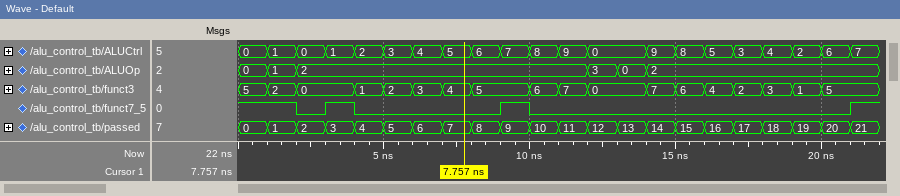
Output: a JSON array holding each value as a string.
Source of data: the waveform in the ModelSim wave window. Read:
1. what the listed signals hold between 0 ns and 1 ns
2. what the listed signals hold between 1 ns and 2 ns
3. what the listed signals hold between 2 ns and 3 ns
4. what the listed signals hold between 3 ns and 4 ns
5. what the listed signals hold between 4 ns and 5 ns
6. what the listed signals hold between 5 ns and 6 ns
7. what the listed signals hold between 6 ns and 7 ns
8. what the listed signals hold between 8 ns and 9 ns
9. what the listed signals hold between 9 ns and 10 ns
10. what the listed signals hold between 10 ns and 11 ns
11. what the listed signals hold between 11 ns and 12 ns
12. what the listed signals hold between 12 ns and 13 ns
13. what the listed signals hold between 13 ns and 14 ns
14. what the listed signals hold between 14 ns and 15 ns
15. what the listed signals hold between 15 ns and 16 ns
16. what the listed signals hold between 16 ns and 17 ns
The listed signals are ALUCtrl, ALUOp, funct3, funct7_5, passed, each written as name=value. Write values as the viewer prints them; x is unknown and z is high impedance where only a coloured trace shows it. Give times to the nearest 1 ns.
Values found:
["ALUCtrl=0, ALUOp=0, funct3=5, funct7_5=1, passed=0", "ALUCtrl=1, ALUOp=1, funct3=2, funct7_5=1, passed=1", "ALUCtrl=0, ALUOp=2, funct3=0, funct7_5=0, passed=2", "ALUCtrl=1, ALUOp=2, funct3=0, funct7_5=1, passed=3", "ALUCtrl=2, ALUOp=2, funct3=1, funct7_5=0, passed=4", "ALUCtrl=3, ALUOp=2, funct3=2, funct7_5=0, passed=5", "ALUCtrl=4, ALUOp=2, funct3=3, funct7_5=0, passed=6", "ALUCtrl=6, ALUOp=2, funct3=5, funct7_5=0, passed=8", "ALUCtrl=7, ALUOp=2, funct3=5, funct7_5=1, passed=9", "ALUCtrl=8, ALUOp=2, funct3=6, funct7_5=0, passed=10", "ALUCtrl=9, ALUOp=2, funct3=7, funct7_5=0, passed=11", "ALUCtrl=0, ALUOp=3, funct3=0, funct7_5=0, passed=12", "ALUCtrl=0, ALUOp=0, funct3=0, funct7_5=0, passed=13", "ALUCtrl=9, ALUOp=2, funct3=7, funct7_5=0, passed=14", "ALUCtrl=8, ALUOp=2, funct3=6, funct7_5=0, passed=15", "ALUCtrl=5, ALUOp=2, funct3=4, funct7_5=0, passed=16"]
